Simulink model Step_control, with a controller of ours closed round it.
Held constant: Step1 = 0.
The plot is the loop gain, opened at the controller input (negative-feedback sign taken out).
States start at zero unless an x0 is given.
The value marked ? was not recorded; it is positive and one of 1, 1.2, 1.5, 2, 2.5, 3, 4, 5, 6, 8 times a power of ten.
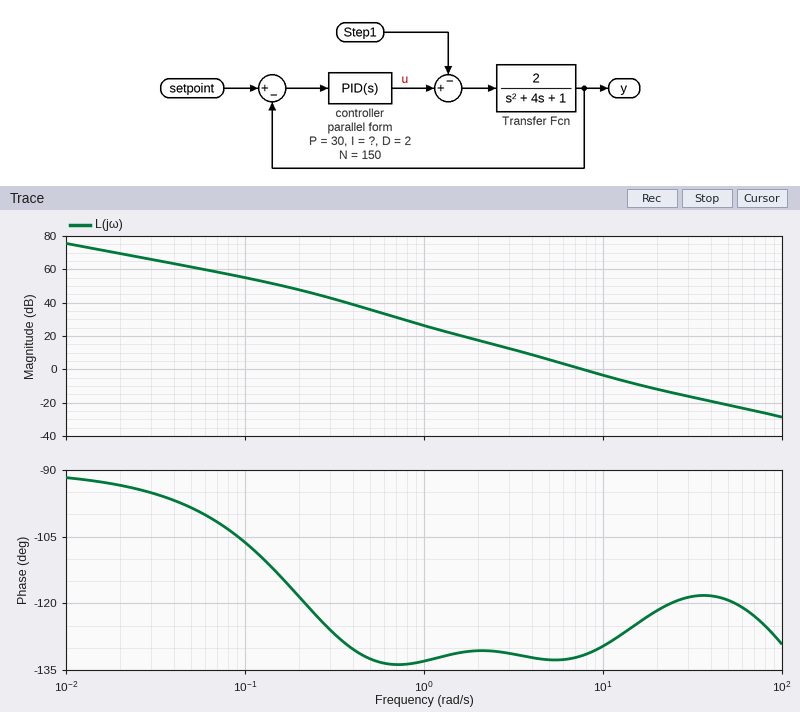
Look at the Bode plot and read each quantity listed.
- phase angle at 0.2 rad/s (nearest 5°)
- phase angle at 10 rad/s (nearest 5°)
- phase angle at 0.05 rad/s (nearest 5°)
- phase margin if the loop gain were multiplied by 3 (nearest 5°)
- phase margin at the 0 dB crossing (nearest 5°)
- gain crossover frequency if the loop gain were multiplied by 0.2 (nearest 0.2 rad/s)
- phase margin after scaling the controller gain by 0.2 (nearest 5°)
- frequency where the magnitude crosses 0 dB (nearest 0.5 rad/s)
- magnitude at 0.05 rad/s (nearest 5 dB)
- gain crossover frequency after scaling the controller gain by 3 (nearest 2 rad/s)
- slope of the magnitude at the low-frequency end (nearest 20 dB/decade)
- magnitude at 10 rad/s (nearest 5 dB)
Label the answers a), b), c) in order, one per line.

a) -120°
b) -130°
c) -100°
d) 55°
e) 50°
f) 2.6 rad/s
g) 50°
h) 7.5 rad/s
i) 60 dB
j) 16 rad/s
k) -20 dB/decade
l) -5 dB
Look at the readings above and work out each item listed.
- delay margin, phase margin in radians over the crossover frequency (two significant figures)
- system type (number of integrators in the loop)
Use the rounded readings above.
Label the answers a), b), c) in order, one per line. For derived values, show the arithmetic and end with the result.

a) 50 × π / 180 / 7.5 = 0.12 s
b) 1
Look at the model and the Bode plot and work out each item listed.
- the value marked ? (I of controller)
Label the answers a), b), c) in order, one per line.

a) 30
